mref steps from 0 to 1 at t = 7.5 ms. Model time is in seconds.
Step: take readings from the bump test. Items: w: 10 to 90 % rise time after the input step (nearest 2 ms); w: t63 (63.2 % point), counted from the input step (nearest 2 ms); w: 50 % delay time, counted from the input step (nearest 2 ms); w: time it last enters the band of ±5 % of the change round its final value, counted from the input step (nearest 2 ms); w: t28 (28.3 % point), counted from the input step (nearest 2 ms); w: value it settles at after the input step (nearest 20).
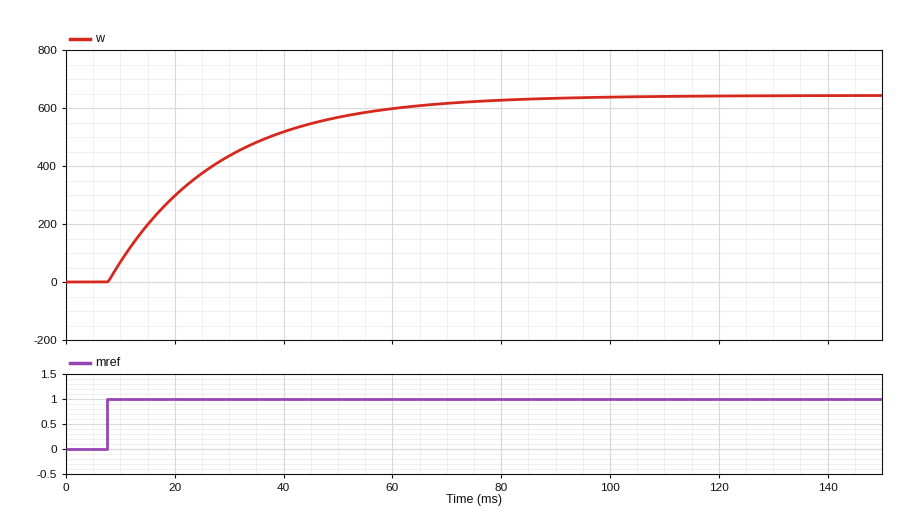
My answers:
44 ms
20 ms
14 ms
60 ms
6 ms
640
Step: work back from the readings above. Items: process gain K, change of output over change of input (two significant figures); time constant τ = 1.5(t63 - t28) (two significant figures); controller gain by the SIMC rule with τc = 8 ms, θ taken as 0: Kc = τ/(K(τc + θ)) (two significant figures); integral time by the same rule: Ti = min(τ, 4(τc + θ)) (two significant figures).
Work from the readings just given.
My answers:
640
21 ms
0.0041
21 ms
